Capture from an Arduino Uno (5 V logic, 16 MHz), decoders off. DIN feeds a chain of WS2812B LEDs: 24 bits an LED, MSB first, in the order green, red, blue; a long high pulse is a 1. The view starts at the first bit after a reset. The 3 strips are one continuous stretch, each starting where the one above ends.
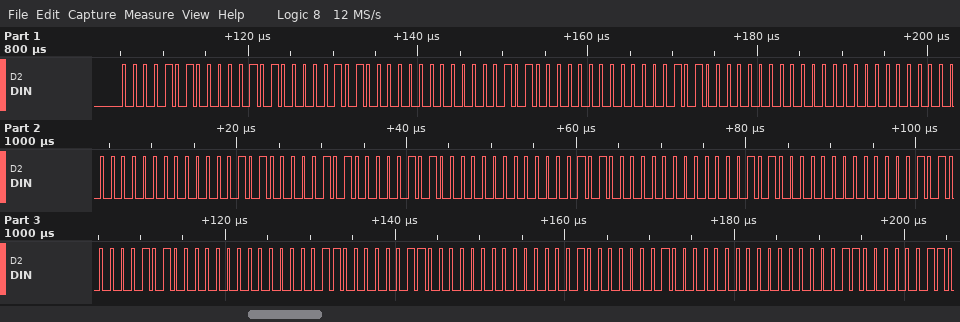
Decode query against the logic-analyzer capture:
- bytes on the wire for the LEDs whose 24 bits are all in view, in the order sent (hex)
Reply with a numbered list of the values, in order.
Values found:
1. 0A 0A 0A 00 0A 00 0A 00 00 00 00 0A 0A 0A 00 0A 00 0A 00 0A 0A 00 06 06 00 04 04 00 03 03
